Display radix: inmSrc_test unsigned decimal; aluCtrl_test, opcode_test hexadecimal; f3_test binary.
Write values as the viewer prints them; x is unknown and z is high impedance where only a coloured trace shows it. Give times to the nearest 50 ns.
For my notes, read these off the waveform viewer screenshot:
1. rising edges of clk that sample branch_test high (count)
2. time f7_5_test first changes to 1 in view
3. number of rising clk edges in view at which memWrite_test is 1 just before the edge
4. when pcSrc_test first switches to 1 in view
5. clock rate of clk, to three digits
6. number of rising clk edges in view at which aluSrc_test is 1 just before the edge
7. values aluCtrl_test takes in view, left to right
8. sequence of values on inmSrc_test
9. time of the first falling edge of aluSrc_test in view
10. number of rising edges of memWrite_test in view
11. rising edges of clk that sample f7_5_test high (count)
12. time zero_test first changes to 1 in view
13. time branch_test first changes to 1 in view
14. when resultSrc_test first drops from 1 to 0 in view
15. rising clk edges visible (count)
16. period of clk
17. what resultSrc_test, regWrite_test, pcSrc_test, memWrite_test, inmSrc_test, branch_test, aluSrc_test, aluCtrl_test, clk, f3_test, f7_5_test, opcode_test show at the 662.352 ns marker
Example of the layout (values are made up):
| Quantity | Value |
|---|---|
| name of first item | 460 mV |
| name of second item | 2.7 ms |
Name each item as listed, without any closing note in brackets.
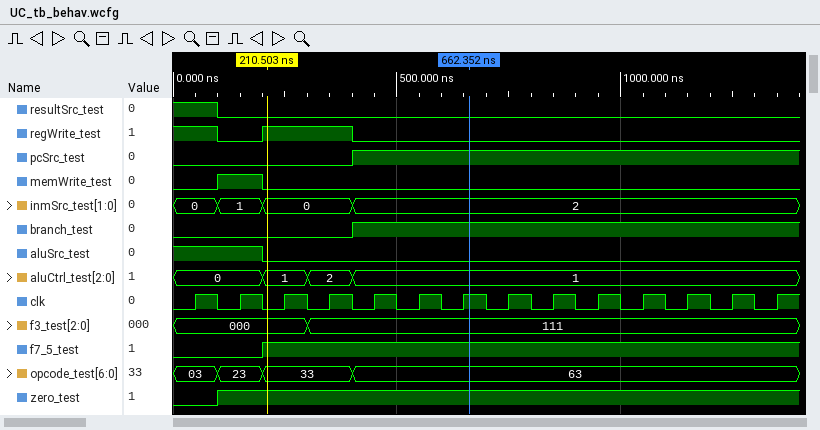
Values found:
| Quantity | Value |
|---|---|
| rising edges of clk that sample branch_test high | 10 |
| time f7_5_test first changes to 1 in view | 200 ns |
| number of rising clk edges in view at which memWrite_test is 1 just before the edge | 1 |
| when pcSrc_test first switches to 1 in view | 400 ns |
| clock rate of clk, to three digits | 10.0 MHz |
| number of rising clk edges in view at which aluSrc_test is 1 just before the edge | 2 |
| values aluCtrl_test takes in view, left to right | 0, 1, 2, 1 |
| sequence of values on inmSrc_test | 0, 1, 0, 2 |
| time of the first falling edge of aluSrc_test in view | 200 ns |
| number of rising edges of memWrite_test in view | 1 |
| rising edges of clk that sample f7_5_test high | 12 |
| time zero_test first changes to 1 in view | 100 ns |
| time branch_test first changes to 1 in view | 400 ns |
| when resultSrc_test first drops from 1 to 0 in view | 100 ns |
| rising clk edges visible | 14 |
| period of clk | 100 ns |
| what resultSrc_test, regWrite_test, pcSrc_test, memWrite_test, inmSrc_test, branch_test, aluSrc_test, aluCtrl_test, clk, f3_test, f7_5_test, opcode_test show at the 662.352 ns marker | resultSrc_test=0, regWrite_test=0, pcSrc_test=1, memWrite_test=0, inmSrc_test=2, branch_test=1, aluSrc_test=0, aluCtrl_test=1, clk=1, f3_test=111, f7_5_test=1, opcode_test=63 |
